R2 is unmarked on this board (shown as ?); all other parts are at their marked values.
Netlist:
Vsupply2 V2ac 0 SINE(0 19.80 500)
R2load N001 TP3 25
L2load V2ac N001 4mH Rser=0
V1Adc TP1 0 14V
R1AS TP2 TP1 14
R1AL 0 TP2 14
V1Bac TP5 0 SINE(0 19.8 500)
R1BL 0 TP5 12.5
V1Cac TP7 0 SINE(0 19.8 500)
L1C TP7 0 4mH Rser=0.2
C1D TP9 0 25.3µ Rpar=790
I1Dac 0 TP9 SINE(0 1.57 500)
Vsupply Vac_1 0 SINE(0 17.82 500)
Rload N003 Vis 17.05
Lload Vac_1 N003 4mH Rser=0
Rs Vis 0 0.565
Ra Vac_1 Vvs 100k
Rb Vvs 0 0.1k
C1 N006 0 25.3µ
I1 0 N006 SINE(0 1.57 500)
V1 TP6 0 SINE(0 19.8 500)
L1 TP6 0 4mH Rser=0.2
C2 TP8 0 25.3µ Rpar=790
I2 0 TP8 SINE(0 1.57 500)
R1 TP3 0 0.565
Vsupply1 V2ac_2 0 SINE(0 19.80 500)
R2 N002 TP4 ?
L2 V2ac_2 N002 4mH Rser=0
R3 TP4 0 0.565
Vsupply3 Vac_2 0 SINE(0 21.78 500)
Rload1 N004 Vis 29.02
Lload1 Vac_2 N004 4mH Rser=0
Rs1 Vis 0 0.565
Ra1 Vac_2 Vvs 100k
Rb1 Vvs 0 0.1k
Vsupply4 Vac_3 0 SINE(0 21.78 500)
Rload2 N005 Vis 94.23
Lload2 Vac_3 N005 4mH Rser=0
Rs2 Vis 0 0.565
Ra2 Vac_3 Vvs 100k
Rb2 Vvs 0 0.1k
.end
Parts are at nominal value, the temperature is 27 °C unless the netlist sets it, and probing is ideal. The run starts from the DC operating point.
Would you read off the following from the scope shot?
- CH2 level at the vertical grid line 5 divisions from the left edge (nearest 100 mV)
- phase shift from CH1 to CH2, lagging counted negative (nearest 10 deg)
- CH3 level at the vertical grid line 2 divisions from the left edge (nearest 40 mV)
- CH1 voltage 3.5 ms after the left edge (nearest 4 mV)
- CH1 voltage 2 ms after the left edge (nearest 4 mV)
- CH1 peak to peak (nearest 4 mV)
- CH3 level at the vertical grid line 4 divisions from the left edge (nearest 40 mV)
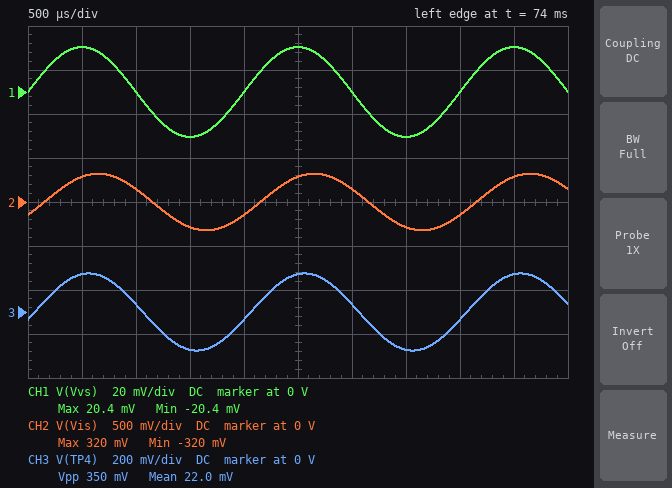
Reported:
300 mV
-30 deg
40 mV
-20 mV
0 V
40 mV
-40 mV
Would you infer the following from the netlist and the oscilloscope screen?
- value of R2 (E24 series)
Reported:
62 Ω
